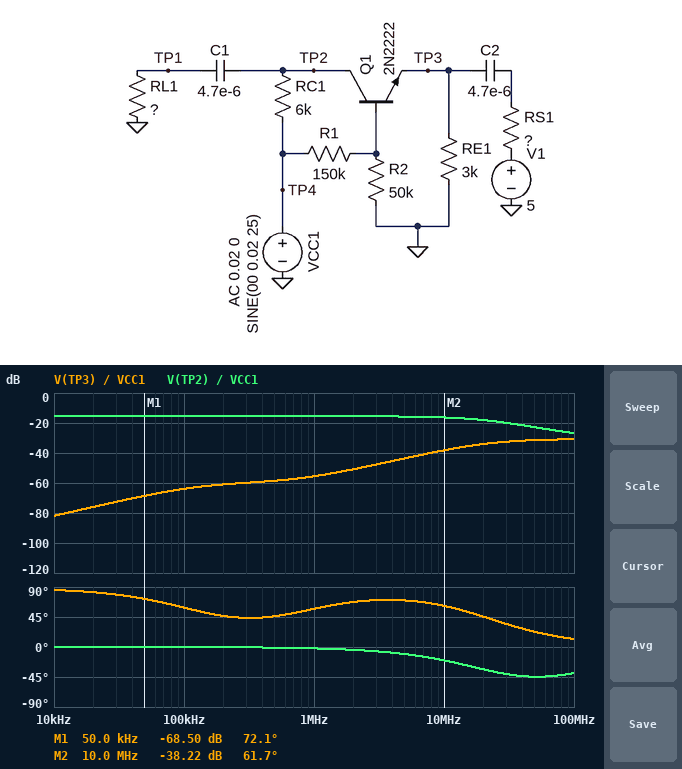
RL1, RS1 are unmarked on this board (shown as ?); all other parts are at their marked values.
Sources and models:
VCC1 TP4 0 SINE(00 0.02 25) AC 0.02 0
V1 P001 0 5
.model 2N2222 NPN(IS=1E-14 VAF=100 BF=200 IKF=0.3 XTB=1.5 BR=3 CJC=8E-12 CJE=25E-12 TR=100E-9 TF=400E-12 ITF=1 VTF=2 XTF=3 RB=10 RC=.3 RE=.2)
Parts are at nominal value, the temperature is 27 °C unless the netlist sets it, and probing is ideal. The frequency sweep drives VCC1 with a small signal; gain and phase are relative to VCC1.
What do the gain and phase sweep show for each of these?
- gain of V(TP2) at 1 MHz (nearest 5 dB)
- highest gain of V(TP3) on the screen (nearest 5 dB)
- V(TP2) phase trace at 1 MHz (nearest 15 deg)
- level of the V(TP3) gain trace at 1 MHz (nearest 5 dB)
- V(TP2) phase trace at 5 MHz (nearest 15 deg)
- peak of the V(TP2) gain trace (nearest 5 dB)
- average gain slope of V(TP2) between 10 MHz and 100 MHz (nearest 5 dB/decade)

-15 dB
-30 dB
0 deg
-55 dB
-15 deg
-15 dB
-10 dB/decade
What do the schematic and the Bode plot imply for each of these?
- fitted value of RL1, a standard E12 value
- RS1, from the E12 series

1.2 kΩ
220 Ω
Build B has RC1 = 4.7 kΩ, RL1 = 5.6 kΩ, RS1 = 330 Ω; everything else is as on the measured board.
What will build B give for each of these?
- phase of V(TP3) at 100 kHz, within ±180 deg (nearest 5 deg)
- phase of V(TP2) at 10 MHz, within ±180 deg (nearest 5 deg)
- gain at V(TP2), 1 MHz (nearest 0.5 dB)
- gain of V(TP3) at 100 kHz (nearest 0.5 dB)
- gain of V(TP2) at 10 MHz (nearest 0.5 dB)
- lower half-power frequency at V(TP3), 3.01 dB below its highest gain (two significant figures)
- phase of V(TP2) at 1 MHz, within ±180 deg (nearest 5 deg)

75 deg
-40 deg
-5.5 dB
-60.0 dB
-8.5 dB
9.2 MHz
-5 deg
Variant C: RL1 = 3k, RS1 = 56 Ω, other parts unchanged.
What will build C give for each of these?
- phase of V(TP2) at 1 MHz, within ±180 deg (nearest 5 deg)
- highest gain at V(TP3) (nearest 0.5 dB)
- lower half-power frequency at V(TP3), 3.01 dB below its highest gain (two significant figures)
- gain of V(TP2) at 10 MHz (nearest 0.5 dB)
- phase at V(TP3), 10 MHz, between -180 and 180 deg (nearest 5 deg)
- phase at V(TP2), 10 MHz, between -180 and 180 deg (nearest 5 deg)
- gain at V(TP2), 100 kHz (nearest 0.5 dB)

-5 deg
-40.5 dB
13 MHz
-11.5 dB
50 deg
-35 deg
-9.5 dB
